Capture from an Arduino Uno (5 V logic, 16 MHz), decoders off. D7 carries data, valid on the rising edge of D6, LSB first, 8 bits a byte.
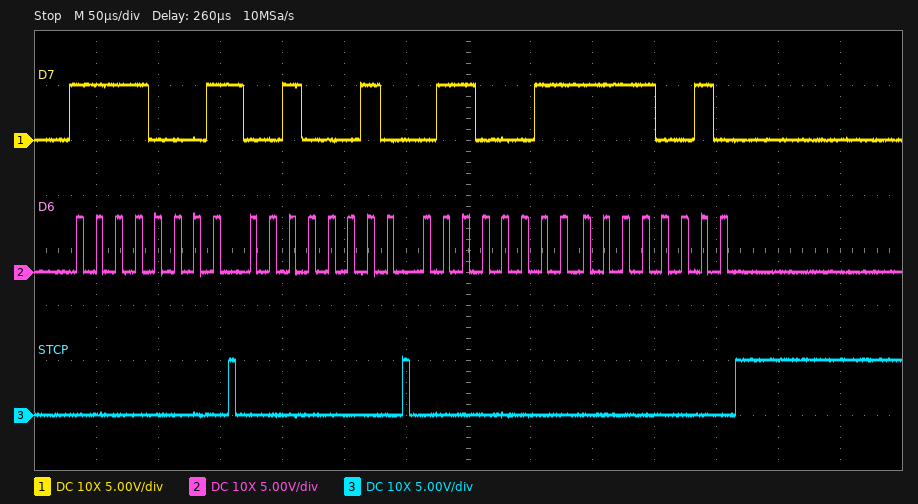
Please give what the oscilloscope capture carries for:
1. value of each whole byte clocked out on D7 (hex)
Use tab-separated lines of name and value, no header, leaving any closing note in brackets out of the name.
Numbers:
value of each whole byte clocked out on D7	8F 44 C6 4F
